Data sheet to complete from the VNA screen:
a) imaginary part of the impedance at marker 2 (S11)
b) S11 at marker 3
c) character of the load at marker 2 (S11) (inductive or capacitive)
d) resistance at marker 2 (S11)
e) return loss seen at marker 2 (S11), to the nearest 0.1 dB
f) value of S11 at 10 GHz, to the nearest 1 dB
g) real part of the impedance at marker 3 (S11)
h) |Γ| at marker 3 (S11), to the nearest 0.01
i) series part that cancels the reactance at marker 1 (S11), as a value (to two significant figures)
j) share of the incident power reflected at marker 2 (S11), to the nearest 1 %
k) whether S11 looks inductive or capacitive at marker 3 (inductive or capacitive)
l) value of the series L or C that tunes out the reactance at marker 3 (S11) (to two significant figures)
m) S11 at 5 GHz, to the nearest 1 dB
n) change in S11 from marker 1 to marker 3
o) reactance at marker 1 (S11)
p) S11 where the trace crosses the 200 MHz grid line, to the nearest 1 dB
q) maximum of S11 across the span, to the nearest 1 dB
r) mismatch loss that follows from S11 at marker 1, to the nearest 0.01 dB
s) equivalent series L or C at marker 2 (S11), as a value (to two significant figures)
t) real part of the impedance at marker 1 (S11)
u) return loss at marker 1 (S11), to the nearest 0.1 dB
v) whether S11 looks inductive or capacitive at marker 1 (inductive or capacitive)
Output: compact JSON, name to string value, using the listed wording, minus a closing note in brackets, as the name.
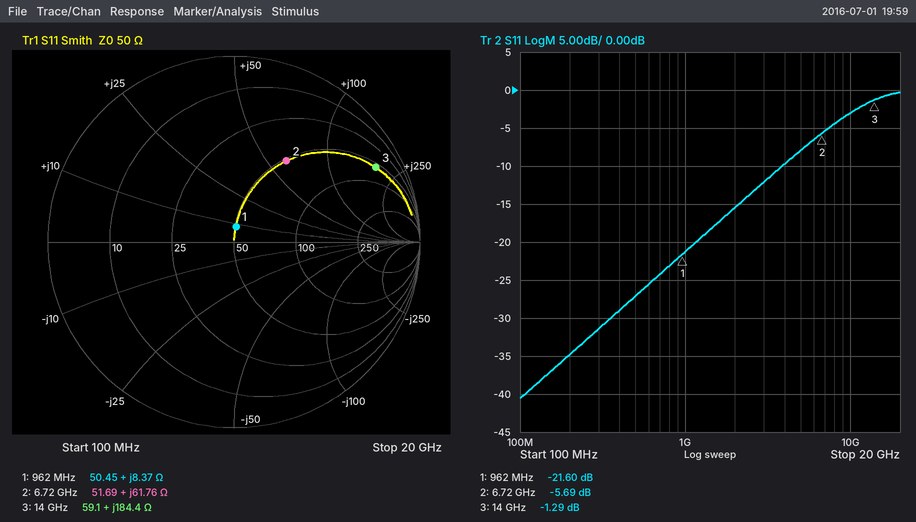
{"imaginary part of the impedance at marker 2": "+61.76 Ω", "S11 at marker 3": "-1.29 dB", "character of the load at marker 2 (S11)": "inductive", "resistance at marker 2": "51.69 Ω", "return loss seen at marker 2 (S11), to the nearest 0.1 dB": "5.7 dB", "value of S11 at 10 GHz, to the nearest 1 dB": "-3 dB", "real part of the impedance at marker 3": "59.1 Ω", "|Γ| at marker 3 (S11), to the nearest 0.01": "0.86", "series part that cancels the reactance at marker 1 (S11), as a value": "20 pF", "share of the incident power reflected at marker 2 (S11), to the nearest 1 %": "27 %", "whether S11 looks inductive or capacitive at marker 3": "inductive", "value of the series L or C that tunes out the reactance at marker 3 (S11)": "62 fF", "S11 at 5 GHz, to the nearest 1 dB": "-8 dB", "change in S11 from marker 1 to marker 3": "20.31 dB", "reactance at marker 1": "+8.37 Ω", "S11 where the trace crosses the 200 MHz grid line, to the nearest 1 dB": "-35 dB", "maximum of S11 across the span, to the nearest 1 dB": "0 dB", "mismatch loss that follows from S11 at marker 1, to the nearest 0.01 dB": "0.03 dB", "equivalent series L or C at marker 2 (S11), as a value": "1.5 nH", "real part of the impedance at marker 1": "50.45 Ω", "return loss at marker 1 (S11), to the nearest 0.1 dB": "21.6 dB", "whether S11 looks inductive or capacitive at marker 1": "inductive"}
